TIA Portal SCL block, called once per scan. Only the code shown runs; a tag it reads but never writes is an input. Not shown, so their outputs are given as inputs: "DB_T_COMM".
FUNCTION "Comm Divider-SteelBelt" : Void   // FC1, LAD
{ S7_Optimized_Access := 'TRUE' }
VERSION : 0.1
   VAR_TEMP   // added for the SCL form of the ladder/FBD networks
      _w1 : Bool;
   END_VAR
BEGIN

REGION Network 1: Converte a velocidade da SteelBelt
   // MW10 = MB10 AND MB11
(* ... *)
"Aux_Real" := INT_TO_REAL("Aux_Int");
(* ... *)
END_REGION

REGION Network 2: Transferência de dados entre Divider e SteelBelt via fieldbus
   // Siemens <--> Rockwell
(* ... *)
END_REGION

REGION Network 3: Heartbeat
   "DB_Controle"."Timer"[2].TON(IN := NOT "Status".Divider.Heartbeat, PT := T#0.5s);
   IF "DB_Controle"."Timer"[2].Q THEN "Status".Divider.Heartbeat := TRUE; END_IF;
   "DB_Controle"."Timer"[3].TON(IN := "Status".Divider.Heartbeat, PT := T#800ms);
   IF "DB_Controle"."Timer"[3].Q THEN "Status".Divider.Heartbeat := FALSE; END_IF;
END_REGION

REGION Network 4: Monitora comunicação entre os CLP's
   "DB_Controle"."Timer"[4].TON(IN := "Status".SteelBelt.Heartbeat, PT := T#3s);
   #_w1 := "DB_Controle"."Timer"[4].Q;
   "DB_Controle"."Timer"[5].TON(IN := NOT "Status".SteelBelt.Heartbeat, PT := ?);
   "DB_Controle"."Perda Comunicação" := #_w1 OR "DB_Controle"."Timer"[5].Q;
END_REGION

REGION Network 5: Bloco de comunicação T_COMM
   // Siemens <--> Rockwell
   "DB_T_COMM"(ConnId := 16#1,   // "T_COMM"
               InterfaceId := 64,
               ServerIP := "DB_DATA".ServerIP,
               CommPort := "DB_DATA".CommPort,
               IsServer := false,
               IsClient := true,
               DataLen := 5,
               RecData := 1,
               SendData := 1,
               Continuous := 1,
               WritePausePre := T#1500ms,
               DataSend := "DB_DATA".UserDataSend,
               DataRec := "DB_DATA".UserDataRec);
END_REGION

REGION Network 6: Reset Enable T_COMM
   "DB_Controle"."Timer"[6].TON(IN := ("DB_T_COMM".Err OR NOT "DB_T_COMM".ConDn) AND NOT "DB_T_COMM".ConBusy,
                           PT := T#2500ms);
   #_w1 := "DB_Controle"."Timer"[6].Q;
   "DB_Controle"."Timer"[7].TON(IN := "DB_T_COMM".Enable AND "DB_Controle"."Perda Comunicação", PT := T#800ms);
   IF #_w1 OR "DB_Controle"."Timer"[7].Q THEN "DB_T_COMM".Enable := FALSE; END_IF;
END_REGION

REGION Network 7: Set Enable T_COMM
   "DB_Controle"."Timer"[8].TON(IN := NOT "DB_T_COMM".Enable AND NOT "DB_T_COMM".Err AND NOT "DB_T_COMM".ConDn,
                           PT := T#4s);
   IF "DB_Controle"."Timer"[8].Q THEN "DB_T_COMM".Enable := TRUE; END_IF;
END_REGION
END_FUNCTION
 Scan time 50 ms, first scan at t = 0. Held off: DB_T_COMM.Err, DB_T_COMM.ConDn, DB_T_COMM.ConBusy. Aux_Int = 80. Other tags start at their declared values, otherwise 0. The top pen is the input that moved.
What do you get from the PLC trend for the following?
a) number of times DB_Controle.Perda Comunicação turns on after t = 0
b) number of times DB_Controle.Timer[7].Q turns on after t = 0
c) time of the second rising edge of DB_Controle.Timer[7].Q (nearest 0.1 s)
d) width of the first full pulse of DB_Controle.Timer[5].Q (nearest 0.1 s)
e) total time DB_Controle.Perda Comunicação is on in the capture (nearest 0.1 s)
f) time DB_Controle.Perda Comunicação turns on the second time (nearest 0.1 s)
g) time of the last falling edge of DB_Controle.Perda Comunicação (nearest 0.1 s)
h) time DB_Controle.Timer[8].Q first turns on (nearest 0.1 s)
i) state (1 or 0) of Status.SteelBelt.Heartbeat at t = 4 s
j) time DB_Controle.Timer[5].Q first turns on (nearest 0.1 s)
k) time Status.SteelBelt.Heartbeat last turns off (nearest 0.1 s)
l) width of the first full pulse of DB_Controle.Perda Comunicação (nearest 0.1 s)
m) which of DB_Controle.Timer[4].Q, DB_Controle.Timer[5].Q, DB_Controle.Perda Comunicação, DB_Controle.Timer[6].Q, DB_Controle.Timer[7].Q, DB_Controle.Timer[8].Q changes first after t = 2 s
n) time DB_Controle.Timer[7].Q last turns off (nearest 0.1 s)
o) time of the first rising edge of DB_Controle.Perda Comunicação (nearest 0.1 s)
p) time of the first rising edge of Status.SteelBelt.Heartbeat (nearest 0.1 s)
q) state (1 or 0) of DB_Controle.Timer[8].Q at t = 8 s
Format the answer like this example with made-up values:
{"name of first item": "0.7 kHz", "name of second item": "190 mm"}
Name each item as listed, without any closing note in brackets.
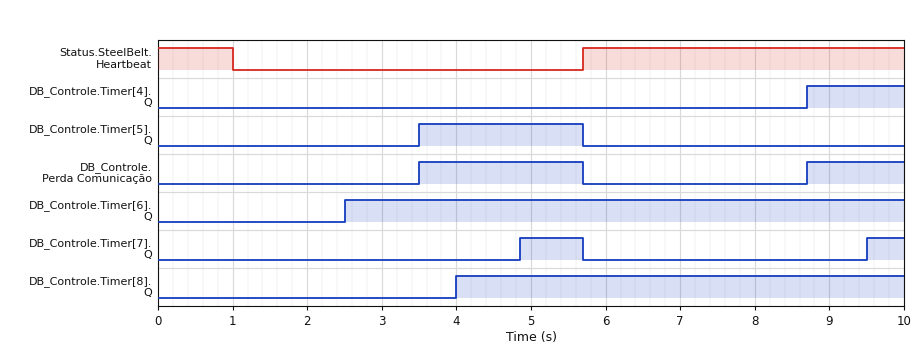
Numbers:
{"number of times DB_Controle.Perda Comunicação turns on after t = 0": "2", "number of times DB_Controle.Timer[7].Q turns on after t = 0": "2", "time of the second rising edge of DB_Controle.Timer[7].Q": "9.5 s", "width of the first full pulse of DB_Controle.Timer[5].Q": "2.2 s", "total time DB_Controle.Perda Comunicação is on in the capture": "3.5 s", "time DB_Controle.Perda Comunicação turns on the second time": "8.7 s", "time of the last falling edge of DB_Controle.Perda Comunicação": "5.7 s", "time DB_Controle.Timer[8].Q first turns on": "4.0 s", "state (1 or 0) of Status.SteelBelt.Heartbeat at t = 4 s": "0", "time DB_Controle.Timer[5].Q first turns on": "3.5 s", "time Status.SteelBelt.Heartbeat last turns off": "1.0 s", "width of the first full pulse of DB_Controle.Perda Comunicação": "2.2 s", "which of DB_Controle.Timer[4].Q, DB_Controle.Timer[5].Q, DB_Controle.Perda Comunicação, DB_Controle.Timer[6].Q, DB_Controle.Timer[7].Q, DB_Controle.Timer[8].Q changes first after t = 2 s": "DB_Controle.Timer[6].Q", "time DB_Controle.Timer[7].Q last turns off": "5.7 s", "time of the first rising edge of DB_Controle.Perda Comunicação": "3.5 s", "time of the first rising edge of Status.SteelBelt.Heartbeat": "5.7 s", "state (1 or 0) of DB_Controle.Timer[8].Q at t = 8 s": "1"}
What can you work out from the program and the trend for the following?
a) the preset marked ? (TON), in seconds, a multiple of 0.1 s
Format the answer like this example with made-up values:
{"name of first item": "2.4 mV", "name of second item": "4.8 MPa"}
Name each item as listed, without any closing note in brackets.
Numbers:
{"the preset marked ? (TON), in seconds, a multiple of 0.1 s": "2.5 s"}
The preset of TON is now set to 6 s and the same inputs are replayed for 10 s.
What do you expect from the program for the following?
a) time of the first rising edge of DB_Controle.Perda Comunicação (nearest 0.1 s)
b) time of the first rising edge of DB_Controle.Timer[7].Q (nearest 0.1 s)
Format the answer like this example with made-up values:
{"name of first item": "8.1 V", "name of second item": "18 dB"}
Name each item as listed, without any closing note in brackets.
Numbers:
{"time of the first rising edge of DB_Controle.Perda Comunicação": "8.7 s", "time of the first rising edge of DB_Controle.Timer[7].Q": "9.5 s"}
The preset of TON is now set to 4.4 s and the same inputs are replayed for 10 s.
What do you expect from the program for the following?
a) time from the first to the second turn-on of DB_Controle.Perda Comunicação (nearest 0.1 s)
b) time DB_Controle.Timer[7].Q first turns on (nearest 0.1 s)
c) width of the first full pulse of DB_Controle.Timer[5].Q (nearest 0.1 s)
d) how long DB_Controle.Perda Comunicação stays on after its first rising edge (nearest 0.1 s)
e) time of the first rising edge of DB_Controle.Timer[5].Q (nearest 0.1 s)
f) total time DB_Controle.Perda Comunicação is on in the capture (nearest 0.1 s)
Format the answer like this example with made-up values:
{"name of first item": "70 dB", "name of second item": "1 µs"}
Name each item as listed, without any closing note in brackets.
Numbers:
{"time from the first to the second turn-on of DB_Controle.Perda Comunicação": "3.3 s", "time DB_Controle.Timer[7].Q first turns on": "9.5 s", "width of the first full pulse of DB_Controle.Timer[5].Q": "0.3 s", "how long DB_Controle.Perda Comunicação stays on after its first rising edge": "0.3 s", "time of the first rising edge of DB_Controle.Timer[5].Q": "5.4 s", "total time DB_Controle.Perda Comunicação is on in the capture": "1.6 s"}
